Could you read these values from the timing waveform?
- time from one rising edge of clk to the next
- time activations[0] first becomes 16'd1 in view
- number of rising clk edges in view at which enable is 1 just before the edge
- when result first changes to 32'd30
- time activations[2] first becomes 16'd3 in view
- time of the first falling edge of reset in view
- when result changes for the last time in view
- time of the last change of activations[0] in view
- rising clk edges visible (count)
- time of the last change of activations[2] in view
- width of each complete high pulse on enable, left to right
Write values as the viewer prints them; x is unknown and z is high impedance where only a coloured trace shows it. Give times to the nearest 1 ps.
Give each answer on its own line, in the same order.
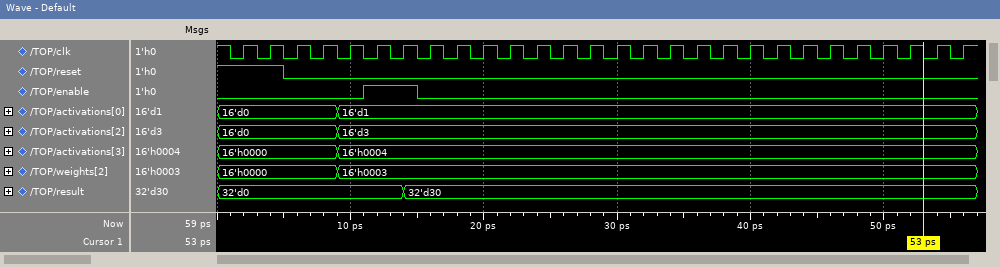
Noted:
2 ps
9 ps
2
14 ps
9 ps
5 ps
14 ps
9 ps
28
9 ps
4 ps
